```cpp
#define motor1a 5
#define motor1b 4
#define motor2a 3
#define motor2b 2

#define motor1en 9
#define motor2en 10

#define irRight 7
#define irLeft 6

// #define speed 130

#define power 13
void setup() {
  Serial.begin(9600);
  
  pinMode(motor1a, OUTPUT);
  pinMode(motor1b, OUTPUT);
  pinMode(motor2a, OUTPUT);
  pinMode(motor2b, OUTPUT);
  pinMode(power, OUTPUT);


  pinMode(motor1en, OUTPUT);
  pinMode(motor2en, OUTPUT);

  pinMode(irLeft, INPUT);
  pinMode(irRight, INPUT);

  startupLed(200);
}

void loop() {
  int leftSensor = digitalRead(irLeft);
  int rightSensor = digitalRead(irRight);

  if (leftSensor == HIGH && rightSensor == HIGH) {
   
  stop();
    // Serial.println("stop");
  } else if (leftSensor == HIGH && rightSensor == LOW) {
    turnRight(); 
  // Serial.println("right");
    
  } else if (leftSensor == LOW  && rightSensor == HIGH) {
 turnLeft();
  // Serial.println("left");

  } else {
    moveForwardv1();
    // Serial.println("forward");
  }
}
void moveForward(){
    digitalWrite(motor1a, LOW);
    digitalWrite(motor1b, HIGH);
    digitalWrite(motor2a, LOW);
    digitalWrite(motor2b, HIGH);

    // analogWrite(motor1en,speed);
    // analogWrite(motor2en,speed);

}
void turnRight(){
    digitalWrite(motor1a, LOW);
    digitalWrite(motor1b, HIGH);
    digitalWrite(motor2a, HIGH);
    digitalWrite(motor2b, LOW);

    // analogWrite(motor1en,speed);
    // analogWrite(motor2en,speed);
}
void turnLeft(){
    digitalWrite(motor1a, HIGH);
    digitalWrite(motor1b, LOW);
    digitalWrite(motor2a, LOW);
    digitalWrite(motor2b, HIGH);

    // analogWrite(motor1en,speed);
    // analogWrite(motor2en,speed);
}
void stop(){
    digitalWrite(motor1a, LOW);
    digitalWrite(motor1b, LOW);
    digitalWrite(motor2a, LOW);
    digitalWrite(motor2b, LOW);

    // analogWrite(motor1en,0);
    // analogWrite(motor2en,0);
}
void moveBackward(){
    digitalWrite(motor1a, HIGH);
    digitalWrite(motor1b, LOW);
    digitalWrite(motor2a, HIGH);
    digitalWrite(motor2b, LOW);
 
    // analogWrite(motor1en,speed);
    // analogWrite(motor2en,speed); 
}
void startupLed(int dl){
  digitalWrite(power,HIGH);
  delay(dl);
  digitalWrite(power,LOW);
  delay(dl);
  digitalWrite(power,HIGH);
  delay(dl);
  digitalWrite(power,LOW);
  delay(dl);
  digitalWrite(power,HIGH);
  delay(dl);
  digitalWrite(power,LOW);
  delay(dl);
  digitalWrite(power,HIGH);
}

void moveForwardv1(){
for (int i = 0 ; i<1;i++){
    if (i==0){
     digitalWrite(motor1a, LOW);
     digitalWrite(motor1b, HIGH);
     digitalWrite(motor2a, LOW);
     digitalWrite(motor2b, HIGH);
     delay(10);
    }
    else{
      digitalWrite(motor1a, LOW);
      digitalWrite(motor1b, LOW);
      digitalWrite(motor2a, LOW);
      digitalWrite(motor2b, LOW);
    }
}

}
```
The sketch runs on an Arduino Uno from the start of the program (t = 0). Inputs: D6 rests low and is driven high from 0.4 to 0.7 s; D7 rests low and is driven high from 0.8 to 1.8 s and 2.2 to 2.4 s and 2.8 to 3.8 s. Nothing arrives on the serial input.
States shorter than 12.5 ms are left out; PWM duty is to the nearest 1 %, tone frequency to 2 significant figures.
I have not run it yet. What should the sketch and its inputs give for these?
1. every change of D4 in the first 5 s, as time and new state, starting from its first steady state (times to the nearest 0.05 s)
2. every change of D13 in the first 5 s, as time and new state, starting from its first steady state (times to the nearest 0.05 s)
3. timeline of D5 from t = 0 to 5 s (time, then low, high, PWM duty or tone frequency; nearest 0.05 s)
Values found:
0 s low; 1.8 s high; 2.2 s low; 2.4 s high; 2.8 s low; 3.8 s high
0 s high; 0.2 s low; 0.4 s high; 0.6 s low; 0.8 s high; 1 s low; 1.2 s high
0 s low; 1.2 s high; 1.8 s low; 2.2 s high; 2.4 s low; 2.8 s high; 3.8 s low
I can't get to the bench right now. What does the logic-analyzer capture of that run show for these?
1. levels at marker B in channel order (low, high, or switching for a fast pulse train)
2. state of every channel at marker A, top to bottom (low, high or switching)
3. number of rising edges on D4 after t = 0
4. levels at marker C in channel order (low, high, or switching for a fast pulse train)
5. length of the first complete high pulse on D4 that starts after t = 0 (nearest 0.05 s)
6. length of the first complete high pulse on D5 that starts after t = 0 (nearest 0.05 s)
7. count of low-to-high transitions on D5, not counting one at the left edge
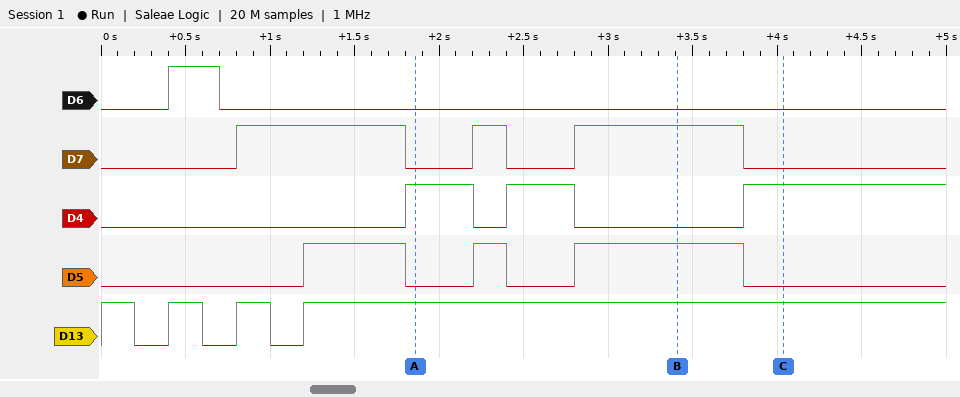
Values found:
D6 low, D7 high, D4 low, D5 high, D13 high
D6 low, D7 low, D4 high, D5 low, D13 high
3
D6 low, D7 low, D4 high, D5 low, D13 high
0.40 s
0.60 s
3
